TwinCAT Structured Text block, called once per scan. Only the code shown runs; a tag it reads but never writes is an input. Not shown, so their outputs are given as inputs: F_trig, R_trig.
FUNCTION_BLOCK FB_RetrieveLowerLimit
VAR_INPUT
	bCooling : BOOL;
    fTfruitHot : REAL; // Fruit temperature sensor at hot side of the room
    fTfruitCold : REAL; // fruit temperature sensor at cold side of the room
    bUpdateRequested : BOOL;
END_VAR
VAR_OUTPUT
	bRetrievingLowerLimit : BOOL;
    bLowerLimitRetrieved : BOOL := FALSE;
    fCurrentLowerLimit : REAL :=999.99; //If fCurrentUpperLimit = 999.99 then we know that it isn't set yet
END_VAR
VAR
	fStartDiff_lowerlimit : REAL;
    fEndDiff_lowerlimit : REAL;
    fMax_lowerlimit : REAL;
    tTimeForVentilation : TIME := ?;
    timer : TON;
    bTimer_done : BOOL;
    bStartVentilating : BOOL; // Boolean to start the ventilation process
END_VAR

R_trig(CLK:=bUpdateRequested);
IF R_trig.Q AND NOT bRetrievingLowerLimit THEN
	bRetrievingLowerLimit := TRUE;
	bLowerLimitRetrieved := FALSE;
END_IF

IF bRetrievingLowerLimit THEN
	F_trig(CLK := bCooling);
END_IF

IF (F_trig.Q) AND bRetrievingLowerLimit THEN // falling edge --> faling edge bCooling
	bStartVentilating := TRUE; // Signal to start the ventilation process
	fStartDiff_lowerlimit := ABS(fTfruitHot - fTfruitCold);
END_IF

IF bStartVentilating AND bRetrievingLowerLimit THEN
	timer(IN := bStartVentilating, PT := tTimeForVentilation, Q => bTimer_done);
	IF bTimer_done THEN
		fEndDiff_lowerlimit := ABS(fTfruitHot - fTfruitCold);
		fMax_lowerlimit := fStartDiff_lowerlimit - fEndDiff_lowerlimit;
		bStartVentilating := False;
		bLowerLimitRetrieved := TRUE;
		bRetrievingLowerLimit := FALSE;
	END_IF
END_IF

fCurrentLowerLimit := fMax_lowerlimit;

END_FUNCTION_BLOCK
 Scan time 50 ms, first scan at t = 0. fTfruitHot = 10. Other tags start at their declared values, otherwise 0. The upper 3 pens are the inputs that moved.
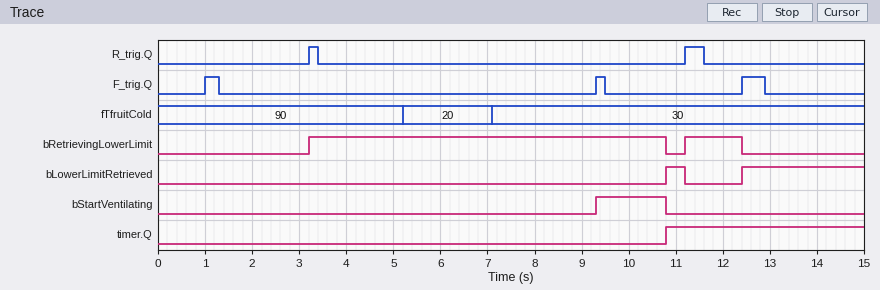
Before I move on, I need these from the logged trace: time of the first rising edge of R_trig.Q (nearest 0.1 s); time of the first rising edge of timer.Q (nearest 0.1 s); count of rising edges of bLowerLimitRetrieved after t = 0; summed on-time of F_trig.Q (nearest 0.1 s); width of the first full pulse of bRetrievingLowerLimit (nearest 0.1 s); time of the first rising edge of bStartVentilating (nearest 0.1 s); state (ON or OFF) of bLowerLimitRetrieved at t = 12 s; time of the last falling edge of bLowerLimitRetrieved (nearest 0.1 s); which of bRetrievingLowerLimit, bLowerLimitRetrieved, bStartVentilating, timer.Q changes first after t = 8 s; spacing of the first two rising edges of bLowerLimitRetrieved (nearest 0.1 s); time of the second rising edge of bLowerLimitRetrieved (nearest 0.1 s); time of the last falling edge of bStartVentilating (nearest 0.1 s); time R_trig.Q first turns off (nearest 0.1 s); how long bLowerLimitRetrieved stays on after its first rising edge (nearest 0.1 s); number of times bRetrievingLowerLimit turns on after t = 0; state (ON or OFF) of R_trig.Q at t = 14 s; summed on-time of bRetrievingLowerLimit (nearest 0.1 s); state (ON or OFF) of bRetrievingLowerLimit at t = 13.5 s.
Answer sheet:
3.2 s
10.8 s
2
1.0 s
7.6 s
9.3 s
OFF
11.2 s
bStartVentilating
1.6 s
12.4 s
10.8 s
3.4 s
0.4 s
2
OFF
8.8 s
OFF
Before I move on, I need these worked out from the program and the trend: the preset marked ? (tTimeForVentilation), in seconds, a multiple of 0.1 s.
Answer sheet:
1.5 s
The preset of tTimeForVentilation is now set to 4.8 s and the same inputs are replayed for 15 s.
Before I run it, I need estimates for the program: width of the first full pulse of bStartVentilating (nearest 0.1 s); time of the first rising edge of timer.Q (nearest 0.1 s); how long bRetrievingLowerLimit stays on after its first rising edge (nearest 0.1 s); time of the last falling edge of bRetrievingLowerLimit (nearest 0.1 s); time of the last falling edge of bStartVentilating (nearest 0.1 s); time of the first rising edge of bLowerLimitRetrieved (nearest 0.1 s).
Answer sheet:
4.8 s
14.1 s
10.9 s
14.1 s
14.1 s
14.1 s
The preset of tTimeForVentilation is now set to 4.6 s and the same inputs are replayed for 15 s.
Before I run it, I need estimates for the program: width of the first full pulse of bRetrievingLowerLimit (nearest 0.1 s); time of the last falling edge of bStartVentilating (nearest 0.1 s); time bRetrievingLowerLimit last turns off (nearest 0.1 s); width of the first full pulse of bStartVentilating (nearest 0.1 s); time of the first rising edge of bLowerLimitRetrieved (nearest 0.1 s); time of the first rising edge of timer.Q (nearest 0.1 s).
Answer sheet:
10.7 s
13.9 s
13.9 s
4.6 s
13.9 s
13.9 s
